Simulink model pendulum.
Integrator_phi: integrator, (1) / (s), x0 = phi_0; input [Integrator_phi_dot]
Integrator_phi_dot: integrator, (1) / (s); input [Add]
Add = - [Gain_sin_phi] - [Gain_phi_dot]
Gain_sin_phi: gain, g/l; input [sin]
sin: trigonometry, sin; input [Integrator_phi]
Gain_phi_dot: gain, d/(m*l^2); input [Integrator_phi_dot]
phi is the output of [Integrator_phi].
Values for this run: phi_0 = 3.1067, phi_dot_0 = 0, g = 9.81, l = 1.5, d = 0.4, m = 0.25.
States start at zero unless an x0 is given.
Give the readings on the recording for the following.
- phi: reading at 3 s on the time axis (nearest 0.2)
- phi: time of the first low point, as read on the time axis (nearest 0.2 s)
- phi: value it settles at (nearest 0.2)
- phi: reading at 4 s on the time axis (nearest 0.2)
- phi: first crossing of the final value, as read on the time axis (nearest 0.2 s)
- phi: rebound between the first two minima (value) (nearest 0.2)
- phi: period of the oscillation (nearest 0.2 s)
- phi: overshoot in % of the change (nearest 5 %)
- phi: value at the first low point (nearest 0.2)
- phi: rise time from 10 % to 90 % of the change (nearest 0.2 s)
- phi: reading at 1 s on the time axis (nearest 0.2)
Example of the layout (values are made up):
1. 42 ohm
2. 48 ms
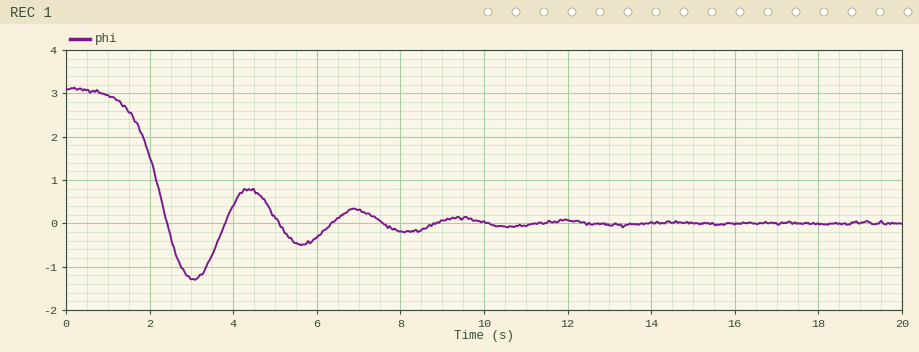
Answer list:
1. -1.2
2. 3.0 s
3. 0.0
4. 0.4
5. 2.4 s
6. 0.8
7. 2.6 s
8. 40 %
9. -1.2
10. 1.0 s
11. 3.0
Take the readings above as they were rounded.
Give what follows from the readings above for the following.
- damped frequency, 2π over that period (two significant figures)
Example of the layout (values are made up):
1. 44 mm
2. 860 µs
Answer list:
1. 2.4 rad/s
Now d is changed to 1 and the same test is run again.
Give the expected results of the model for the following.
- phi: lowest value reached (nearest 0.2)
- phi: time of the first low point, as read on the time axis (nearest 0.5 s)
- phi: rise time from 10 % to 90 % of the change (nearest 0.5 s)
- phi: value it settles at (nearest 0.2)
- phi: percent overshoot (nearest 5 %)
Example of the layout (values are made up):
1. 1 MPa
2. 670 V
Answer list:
1. -0.6
2. 3.5 s
3. 1.5 s
4. 0.0
5. 15 %
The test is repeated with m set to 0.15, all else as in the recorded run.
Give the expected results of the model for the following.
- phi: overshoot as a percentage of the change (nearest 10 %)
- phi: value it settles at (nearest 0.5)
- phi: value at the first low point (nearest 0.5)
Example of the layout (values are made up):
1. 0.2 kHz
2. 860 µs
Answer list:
1. 30 %
2. 0.0
3. -1.0
